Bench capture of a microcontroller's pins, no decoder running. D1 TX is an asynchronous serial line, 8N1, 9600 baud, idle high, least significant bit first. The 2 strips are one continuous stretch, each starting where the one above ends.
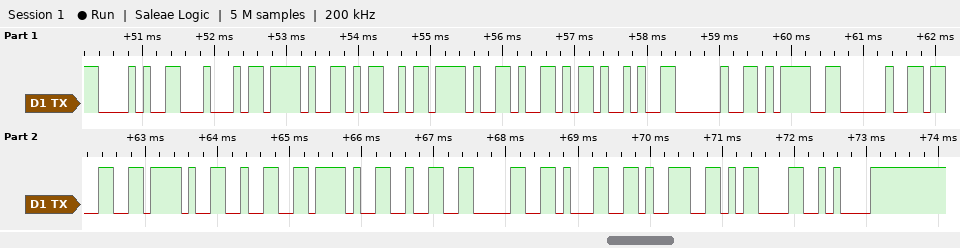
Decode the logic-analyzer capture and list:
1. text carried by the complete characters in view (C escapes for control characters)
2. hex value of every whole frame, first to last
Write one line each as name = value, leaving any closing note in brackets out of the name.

text carried by the complete characters in view = "(D/M/Y) = 3/2/2019\r\n"
hex value of every whole frame, first to last = 0x28 0x44 0x2F 0x4D 0x2F 0x59 0x29 0x20 0x3D 0x20 0x33 0x2F 0x32 0x2F 0x32 0x30 0x31 0x39 0x0D 0x0A
